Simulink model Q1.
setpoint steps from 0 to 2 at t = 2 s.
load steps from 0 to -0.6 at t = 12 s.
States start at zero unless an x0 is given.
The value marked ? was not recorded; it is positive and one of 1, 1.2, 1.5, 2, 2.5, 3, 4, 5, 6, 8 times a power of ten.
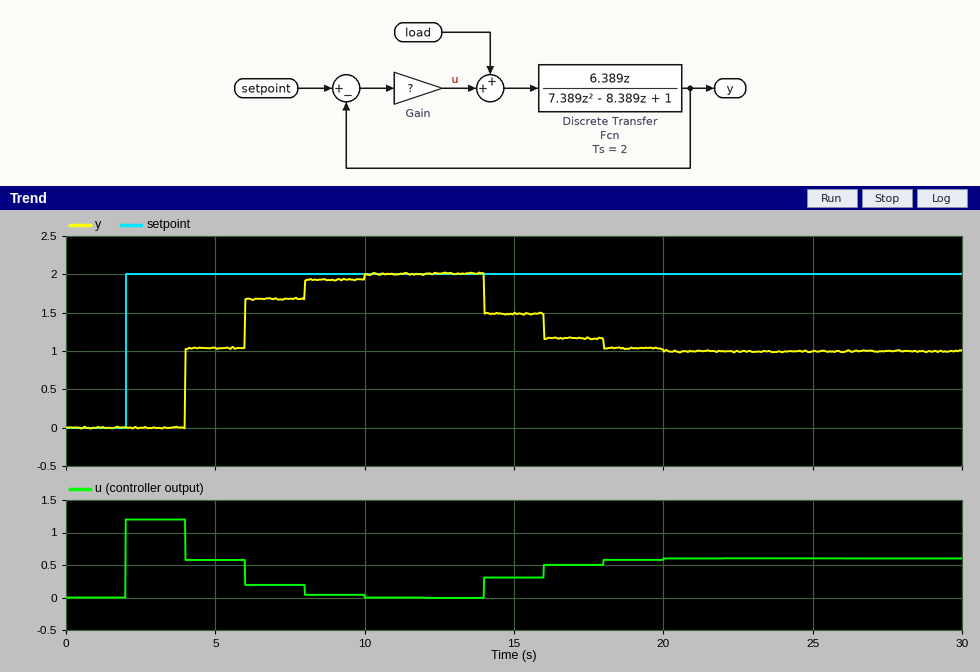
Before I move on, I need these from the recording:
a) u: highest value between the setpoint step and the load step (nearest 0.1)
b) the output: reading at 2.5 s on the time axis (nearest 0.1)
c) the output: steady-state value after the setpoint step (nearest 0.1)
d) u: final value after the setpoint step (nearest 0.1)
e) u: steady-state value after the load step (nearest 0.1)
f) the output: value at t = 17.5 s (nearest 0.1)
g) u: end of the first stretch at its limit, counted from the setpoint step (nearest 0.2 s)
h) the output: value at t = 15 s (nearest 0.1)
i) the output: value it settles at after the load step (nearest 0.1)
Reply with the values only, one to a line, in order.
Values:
1.2
0.0
2.0
0.0
0.6
1.2
2.0 s
1.5
1.0
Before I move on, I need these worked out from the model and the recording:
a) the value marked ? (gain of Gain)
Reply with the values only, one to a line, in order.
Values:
0.6
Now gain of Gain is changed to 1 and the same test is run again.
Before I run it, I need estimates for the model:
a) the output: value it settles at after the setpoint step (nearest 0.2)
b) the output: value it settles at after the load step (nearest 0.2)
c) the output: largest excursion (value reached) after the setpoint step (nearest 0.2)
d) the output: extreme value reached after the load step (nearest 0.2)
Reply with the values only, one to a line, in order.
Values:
2.0
1.4
2.2
1.4
